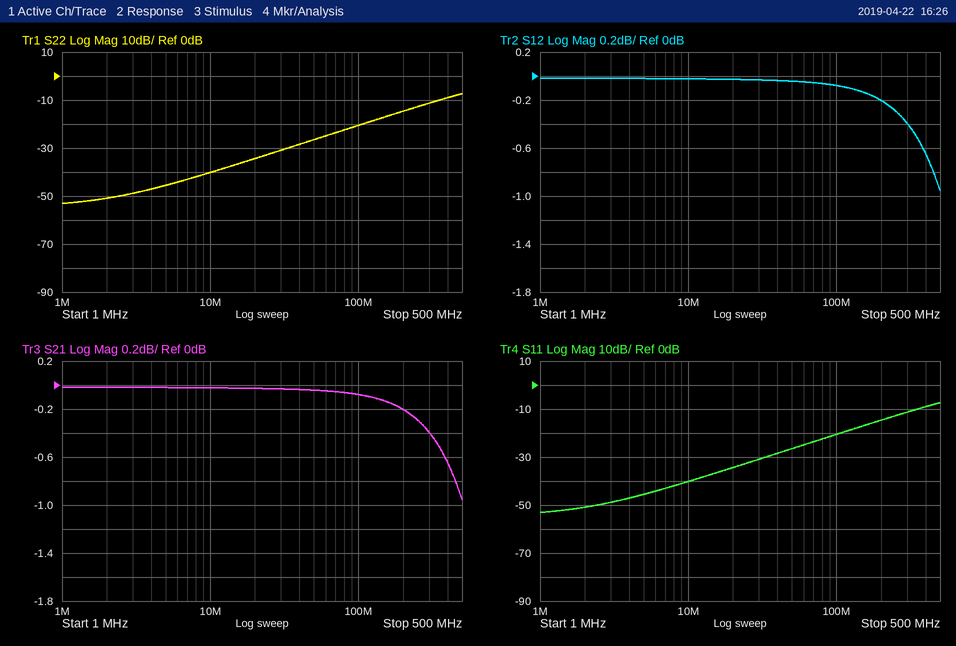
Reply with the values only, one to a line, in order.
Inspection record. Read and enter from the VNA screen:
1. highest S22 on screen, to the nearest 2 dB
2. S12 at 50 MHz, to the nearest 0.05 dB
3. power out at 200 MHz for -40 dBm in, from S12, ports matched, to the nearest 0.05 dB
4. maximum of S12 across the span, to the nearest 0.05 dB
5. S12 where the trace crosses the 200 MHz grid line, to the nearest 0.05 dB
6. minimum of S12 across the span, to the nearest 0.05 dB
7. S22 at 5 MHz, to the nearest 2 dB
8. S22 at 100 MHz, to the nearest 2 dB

-8 dB
-0.05 dB
-40.20 dBm
0.00 dB
-0.20 dB
-0.95 dB
-46 dB
-20 dB
